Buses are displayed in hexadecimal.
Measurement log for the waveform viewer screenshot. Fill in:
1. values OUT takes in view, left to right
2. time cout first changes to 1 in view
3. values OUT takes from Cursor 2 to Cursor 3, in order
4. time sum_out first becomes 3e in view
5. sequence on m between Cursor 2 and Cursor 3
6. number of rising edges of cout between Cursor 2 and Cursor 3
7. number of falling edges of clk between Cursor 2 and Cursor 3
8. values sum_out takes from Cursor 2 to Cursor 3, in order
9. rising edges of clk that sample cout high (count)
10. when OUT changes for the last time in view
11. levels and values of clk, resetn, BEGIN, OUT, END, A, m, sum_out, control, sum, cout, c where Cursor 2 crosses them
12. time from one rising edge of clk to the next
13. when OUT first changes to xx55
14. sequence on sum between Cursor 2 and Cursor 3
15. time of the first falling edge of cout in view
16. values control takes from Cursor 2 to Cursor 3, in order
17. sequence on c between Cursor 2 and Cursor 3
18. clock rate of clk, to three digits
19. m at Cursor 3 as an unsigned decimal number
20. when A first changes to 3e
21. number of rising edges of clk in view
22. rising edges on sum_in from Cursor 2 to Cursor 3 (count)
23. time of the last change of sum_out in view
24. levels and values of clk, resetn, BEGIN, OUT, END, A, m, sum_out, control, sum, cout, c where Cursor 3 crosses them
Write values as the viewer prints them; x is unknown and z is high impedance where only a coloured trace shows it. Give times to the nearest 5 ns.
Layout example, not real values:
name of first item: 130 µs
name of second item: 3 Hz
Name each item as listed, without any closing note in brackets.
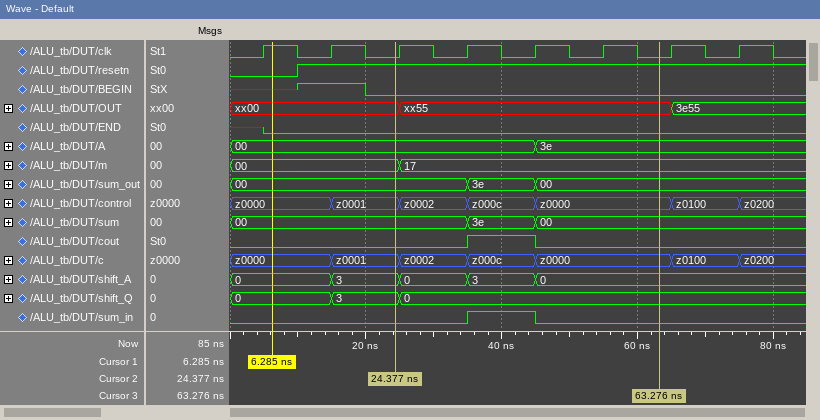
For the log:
values OUT takes in view, left to right: xx00, xx55, 3e55
time cout first changes to 1 in view: 35 ns
values OUT takes from Cursor 2 to Cursor 3, in order: xx00, xx55
time sum_out first becomes 3e in view: 35 ns
sequence on m between Cursor 2 and Cursor 3: 00, 17
number of rising edges of cout between Cursor 2 and Cursor 3: 1
number of falling edges of clk between Cursor 2 and Cursor 3: 4
values sum_out takes from Cursor 2 to Cursor 3, in order: 00, 3e, 00
rising edges of clk that sample cout high: 1
when OUT changes for the last time in view: 65 ns
levels and values of clk, resetn, BEGIN, OUT, END, A, m, sum_out, control, sum, cout, c where Cursor 2 crosses them: clk=0, resetn=1, BEGIN=0, OUT=xx00, END=0, A=00, m=00, sum_out=00, control=z0001, sum=00, cout=0, c=z0001
time from one rising edge of clk to the next: 10 ns
when OUT first changes to xx55: 25 ns
sequence on sum between Cursor 2 and Cursor 3: 00, 3e, 00
time of the first falling edge of cout in view: 45 ns
values control takes from Cursor 2 to Cursor 3, in order: z0001, z0002, z000c, z0000
sequence on c between Cursor 2 and Cursor 3: z0001, z0002, z000c, z0000
clock rate of clk, to three digits: 100 MHz
m at Cursor 3 as an unsigned decimal number: 23
when A first changes to 3e: 45 ns
number of rising edges of clk in view: 8
rising edges on sum_in from Cursor 2 to Cursor 3: 1
time of the last change of sum_out in view: 45 ns
levels and values of clk, resetn, BEGIN, OUT, END, A, m, sum_out, control, sum, cout, c where Cursor 3 crosses them: clk=0, resetn=1, BEGIN=0, OUT=xx55, END=0, A=3e, m=17, sum_out=00, control=z0000, sum=00, cout=0, c=z0000
